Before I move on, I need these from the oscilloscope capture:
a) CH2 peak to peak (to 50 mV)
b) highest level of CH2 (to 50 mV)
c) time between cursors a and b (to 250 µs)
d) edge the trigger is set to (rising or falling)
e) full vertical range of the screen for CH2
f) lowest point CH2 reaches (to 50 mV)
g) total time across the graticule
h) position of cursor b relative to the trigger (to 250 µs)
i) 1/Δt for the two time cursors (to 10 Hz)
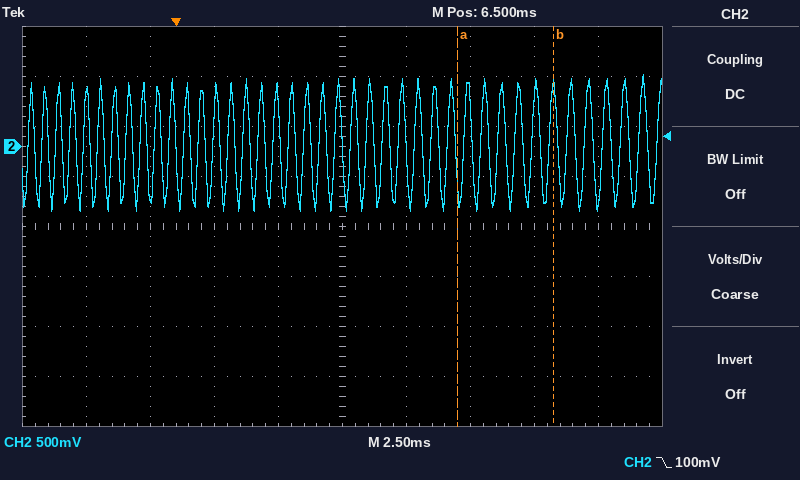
1.35 V
700 mV
3.75 ms
falling
4 V
-650 mV
25 ms
+14.75 ms
270 Hz
